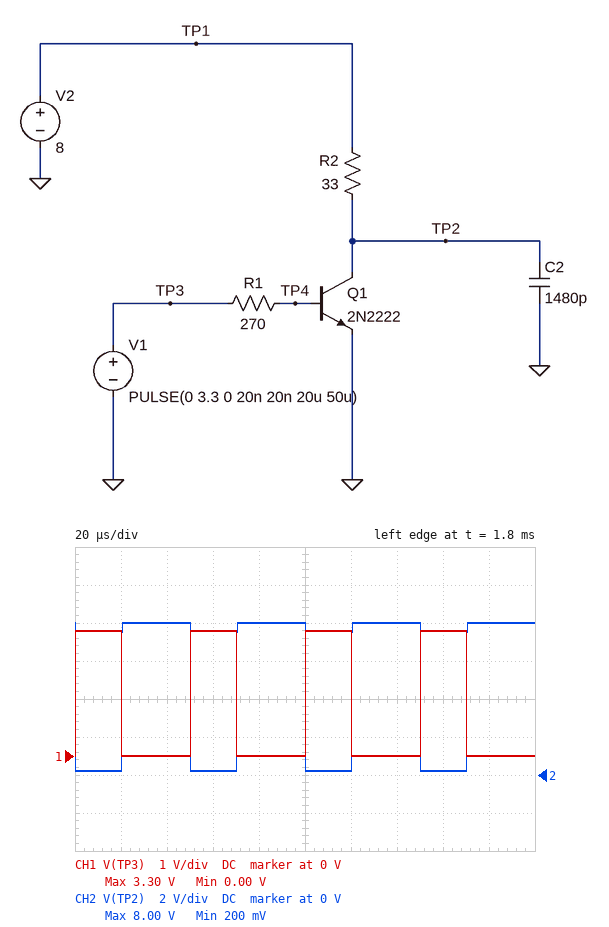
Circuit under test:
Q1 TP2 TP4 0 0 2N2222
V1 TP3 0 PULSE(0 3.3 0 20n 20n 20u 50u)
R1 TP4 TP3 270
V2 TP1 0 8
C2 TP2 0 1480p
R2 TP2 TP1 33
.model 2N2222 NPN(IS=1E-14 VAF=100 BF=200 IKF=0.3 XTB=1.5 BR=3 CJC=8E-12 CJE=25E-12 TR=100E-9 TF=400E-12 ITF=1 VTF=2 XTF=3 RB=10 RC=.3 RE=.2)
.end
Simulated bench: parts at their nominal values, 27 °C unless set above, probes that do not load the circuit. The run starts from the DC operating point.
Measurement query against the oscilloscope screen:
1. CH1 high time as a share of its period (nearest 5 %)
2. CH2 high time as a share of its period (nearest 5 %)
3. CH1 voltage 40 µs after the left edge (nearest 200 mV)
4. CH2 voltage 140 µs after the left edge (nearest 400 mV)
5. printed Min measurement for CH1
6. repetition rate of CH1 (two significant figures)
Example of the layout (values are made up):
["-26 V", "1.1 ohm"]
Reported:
["40 %", "60 %", "0 V", "8.0 V", "0.00 V", "20 kHz"]
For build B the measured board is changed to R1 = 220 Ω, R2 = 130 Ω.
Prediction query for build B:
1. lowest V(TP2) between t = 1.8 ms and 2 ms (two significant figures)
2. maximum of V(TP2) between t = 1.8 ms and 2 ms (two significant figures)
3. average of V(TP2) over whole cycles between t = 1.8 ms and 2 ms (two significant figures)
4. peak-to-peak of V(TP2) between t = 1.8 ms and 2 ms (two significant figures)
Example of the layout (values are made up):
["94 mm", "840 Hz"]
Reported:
["62 mV", "8.0 V", "4.7 V", "7.9 V"]
